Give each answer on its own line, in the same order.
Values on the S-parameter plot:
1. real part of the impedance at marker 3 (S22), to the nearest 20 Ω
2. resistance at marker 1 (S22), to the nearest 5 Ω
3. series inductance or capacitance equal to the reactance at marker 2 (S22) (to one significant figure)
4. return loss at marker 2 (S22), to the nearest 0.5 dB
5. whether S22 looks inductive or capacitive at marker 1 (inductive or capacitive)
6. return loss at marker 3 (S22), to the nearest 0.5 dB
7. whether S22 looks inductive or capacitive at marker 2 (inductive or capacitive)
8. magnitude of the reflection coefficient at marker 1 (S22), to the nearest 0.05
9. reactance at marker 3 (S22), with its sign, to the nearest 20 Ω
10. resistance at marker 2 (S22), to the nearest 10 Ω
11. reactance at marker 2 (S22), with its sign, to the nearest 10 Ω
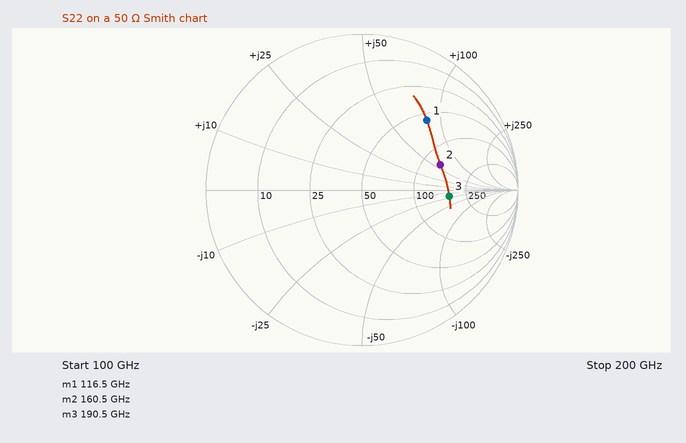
180 Ω
60 Ω
60 pH
5.5 dB
inductive
5.0 dB
inductive
0.60
-20 Ω
130 Ω
+60 Ω
